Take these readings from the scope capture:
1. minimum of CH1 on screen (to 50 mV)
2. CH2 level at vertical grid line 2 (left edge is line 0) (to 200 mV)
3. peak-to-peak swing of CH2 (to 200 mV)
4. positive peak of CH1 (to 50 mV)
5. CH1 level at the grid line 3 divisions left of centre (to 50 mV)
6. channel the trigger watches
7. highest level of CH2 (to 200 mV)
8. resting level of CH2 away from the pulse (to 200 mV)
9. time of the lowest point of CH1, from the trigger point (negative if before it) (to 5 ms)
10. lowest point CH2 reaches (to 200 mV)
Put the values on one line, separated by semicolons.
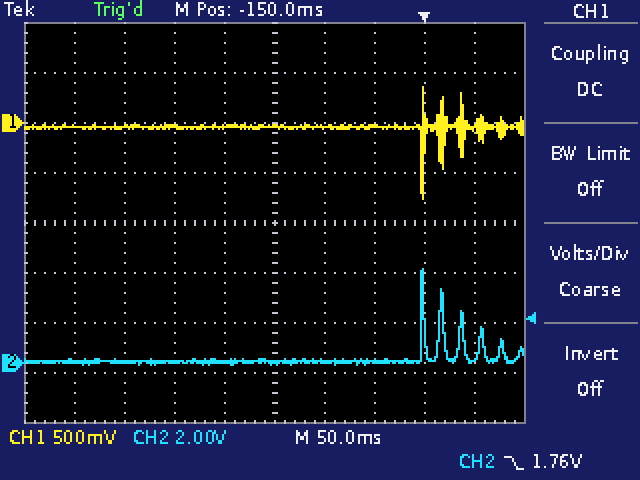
-750 mV; 0.0 V; 3.8 V; 350 mV; -50 mV; CH2; 3.8 V; 0.0 V; 0 ms; 0.0 V
